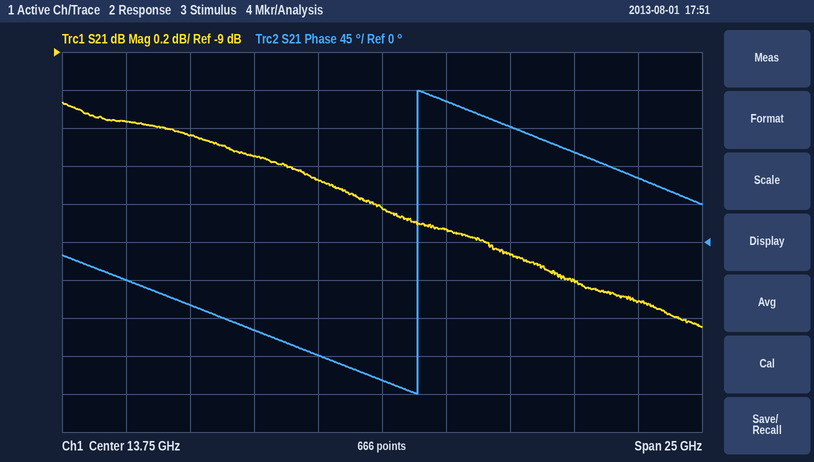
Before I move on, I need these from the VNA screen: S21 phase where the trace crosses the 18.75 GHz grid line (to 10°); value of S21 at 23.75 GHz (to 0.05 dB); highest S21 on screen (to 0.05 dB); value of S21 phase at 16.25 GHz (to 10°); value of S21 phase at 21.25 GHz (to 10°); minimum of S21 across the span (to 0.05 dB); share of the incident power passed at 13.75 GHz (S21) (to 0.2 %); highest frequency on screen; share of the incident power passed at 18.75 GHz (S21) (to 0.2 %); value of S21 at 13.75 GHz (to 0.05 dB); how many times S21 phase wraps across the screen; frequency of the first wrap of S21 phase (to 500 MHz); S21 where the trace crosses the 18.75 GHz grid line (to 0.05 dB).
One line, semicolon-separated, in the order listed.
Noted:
140°; -10.30 dB; -9.25 dB; 170°; 110°; -10.45 dB; 10.4 %; 26.25 GHz; 9.8 %; -9.80 dB; 1; 15.0 GHz; -10.05 dB
